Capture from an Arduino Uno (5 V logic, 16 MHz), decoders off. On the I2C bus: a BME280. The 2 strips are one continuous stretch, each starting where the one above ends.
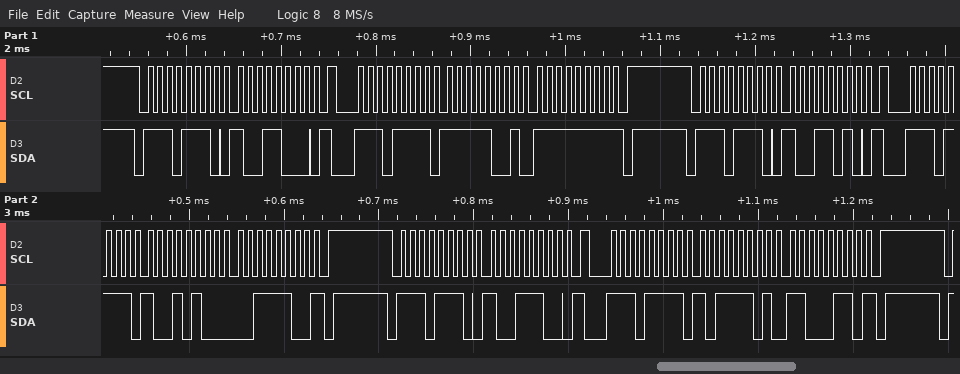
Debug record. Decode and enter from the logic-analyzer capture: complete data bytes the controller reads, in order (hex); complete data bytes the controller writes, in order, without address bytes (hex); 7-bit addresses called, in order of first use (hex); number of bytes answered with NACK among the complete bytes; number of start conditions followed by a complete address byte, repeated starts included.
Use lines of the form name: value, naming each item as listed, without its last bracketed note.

complete data bytes the controller reads, in order: F9 FF 94 3C BD C6
complete data bytes the controller writes, in order, without address bytes: 98 9A 9C
7-bit addresses called, in order of first use: 0x77
number of bytes answered with NACK among the complete bytes: 3
number of start conditions followed by a complete address byte, repeated starts included: 6
